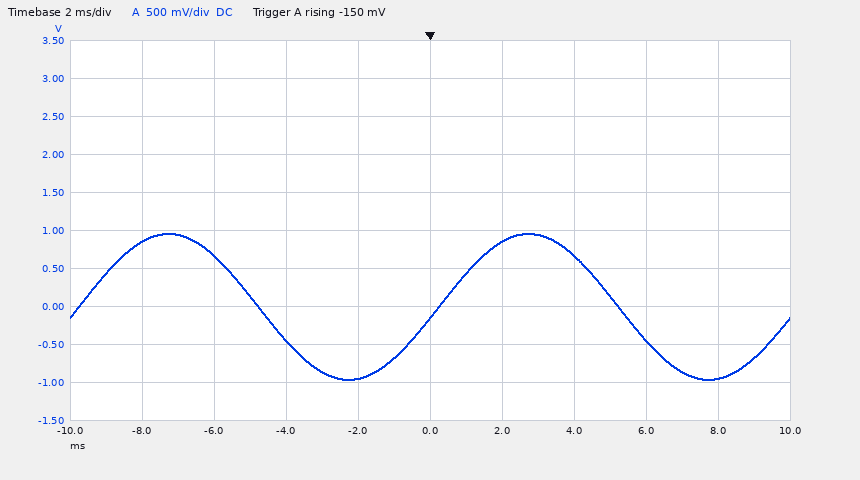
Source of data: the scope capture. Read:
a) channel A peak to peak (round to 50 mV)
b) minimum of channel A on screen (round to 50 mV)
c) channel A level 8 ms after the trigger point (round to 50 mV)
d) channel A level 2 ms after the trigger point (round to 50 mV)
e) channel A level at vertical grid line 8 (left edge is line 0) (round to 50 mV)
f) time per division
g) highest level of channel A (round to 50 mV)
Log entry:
1.90 V
-950 mV
-950 mV
850 mV
-450 mV
2 ms
950 mV
